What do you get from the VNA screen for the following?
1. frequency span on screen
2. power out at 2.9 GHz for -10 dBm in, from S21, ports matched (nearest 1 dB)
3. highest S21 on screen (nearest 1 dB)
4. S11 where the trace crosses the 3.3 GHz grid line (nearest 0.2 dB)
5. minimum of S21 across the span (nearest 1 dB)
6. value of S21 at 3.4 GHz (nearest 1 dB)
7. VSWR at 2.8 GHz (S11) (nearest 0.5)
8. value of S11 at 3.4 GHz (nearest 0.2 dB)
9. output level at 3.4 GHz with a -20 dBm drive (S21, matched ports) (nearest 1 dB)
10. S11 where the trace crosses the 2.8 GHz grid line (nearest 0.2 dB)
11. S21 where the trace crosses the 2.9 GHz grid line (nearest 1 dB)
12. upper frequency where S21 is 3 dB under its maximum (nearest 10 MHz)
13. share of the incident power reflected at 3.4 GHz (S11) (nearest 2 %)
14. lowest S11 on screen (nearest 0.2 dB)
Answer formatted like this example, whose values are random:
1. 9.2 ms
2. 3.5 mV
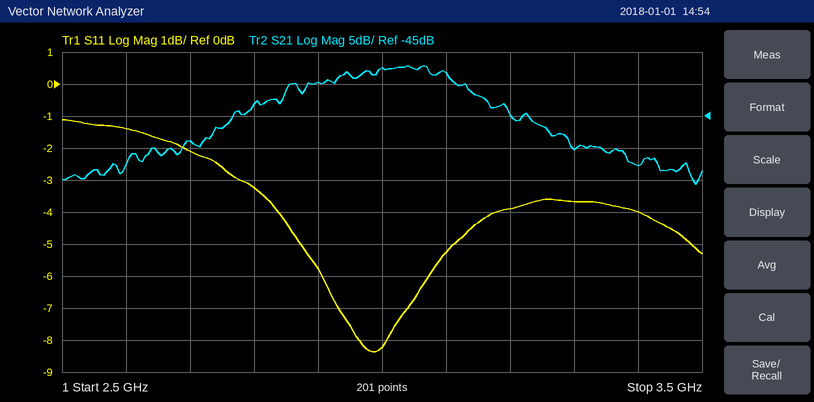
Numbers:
1. 1 GHz
2. -50 dBm
3. -37 dB
4. -3.6 dB
5. -56 dB
6. -53 dB
7. 5.5
8. -4.0 dB
9. -73 dBm
10. -3.2 dB
11. -40 dB
12. 3.12 GHz
13. 40 %
14. -8.4 dB
